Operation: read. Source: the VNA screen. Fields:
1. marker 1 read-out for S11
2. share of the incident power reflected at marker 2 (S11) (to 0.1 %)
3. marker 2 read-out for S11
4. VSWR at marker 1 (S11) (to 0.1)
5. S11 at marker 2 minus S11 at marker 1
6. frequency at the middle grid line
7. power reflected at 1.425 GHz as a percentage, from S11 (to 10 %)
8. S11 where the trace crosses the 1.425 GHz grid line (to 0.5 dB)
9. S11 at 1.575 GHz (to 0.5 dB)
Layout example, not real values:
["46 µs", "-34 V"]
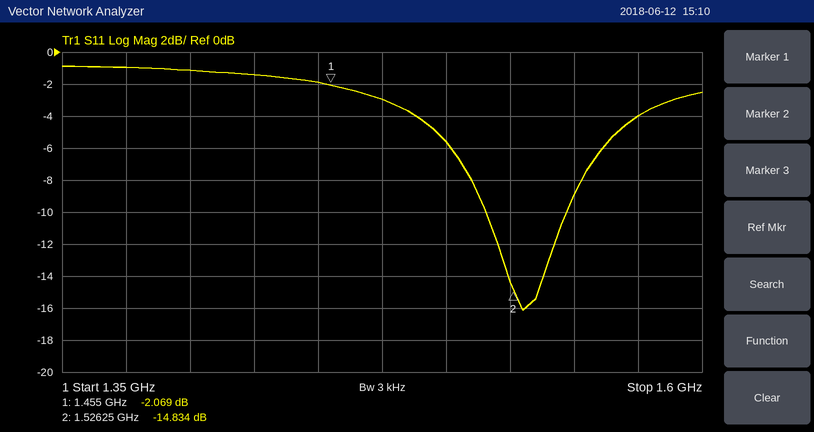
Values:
["-2.069 dB", "3.3 %", "-14.834 dB", "8.4", "-12.765 dB", "1.475 GHz", "70 %", "-1.5 dB", "-4.0 dB"]
